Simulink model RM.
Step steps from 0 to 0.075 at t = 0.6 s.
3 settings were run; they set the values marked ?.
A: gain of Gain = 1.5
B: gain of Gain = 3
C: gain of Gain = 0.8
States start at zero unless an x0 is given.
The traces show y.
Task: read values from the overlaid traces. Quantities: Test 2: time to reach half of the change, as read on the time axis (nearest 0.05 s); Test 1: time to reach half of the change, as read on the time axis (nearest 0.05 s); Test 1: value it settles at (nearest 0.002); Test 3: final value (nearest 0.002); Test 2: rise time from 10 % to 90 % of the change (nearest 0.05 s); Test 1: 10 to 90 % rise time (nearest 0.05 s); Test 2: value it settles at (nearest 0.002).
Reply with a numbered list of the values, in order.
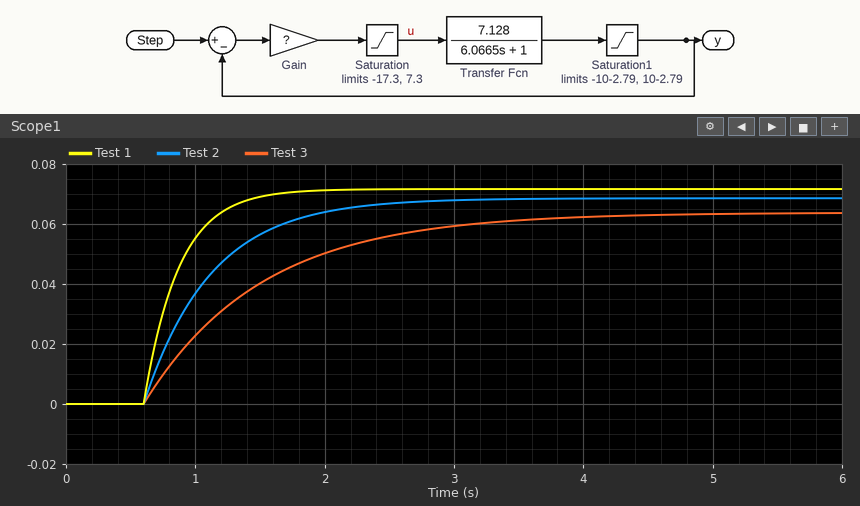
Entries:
1. 0.95 s
2. 0.80 s
3. 0.072
4. 0.064
5. 1.15 s
6. 0.60 s
7. 0.068
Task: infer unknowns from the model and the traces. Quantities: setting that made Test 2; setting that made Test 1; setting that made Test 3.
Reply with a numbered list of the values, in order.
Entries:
1. A
2. B
3. C
